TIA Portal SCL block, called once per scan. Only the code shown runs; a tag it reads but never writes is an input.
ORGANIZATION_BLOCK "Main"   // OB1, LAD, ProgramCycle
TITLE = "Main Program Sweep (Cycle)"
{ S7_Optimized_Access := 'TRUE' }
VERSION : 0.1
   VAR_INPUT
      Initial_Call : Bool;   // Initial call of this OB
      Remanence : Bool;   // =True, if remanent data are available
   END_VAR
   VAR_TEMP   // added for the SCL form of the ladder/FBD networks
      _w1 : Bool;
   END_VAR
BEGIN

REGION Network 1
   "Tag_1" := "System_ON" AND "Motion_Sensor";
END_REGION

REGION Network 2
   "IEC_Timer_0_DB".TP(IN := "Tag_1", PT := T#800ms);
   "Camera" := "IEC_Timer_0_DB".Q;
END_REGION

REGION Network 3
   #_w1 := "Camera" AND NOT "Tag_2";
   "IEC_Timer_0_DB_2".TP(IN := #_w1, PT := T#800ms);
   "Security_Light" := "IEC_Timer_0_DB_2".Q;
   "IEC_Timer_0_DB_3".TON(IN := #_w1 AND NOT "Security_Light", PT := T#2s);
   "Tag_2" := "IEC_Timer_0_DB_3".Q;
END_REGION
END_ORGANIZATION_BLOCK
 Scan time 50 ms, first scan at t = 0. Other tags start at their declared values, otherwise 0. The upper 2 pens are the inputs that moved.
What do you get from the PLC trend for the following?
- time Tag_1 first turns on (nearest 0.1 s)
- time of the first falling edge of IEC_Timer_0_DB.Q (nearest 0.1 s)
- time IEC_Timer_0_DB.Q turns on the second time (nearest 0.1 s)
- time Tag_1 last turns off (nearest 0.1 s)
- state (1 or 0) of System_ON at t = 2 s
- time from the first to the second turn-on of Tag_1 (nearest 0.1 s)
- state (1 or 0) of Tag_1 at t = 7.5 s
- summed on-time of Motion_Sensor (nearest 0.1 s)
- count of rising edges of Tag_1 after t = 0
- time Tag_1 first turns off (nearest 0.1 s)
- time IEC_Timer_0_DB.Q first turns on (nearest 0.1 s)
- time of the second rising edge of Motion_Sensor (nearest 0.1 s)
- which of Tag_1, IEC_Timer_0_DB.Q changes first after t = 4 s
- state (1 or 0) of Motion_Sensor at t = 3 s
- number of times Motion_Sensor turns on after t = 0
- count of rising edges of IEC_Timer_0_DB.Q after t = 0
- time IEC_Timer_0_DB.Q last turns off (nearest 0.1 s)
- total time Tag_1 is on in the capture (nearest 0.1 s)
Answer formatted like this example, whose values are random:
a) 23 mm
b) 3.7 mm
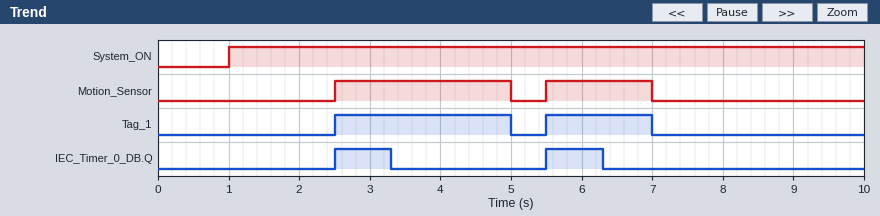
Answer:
a) 2.5 s
b) 3.3 s
c) 5.5 s
d) 7.0 s
e) 1
f) 3.0 s
g) 0
h) 4.0 s
i) 2
j) 5.0 s
k) 2.5 s
l) 5.5 s
m) Tag_1
n) 1
o) 2
p) 2
q) 6.3 s
r) 4.0 s
